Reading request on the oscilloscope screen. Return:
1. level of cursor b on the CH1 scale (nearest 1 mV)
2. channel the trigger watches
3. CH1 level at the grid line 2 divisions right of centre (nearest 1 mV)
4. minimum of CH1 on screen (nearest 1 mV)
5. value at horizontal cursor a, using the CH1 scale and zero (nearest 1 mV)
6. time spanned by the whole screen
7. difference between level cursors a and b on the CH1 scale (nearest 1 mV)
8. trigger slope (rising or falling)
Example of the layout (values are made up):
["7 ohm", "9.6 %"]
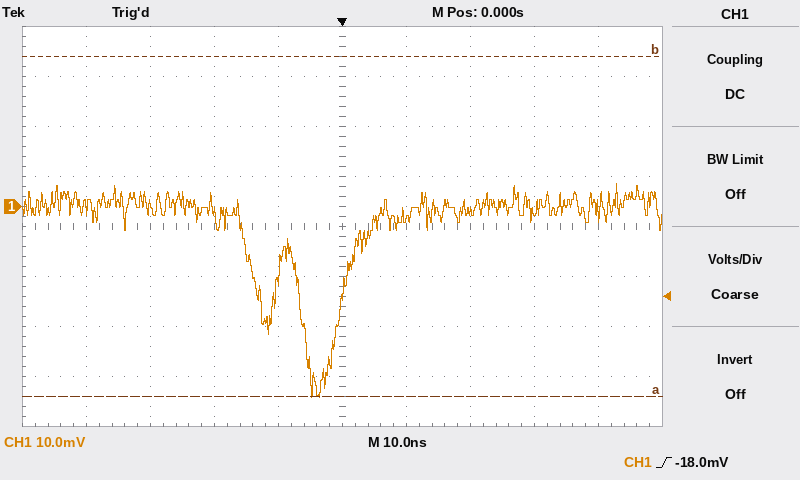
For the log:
["30 mV", "CH1", "-1 mV", "-38 mV", "-38 mV", "100 ns", "68 mV", "rising"]
